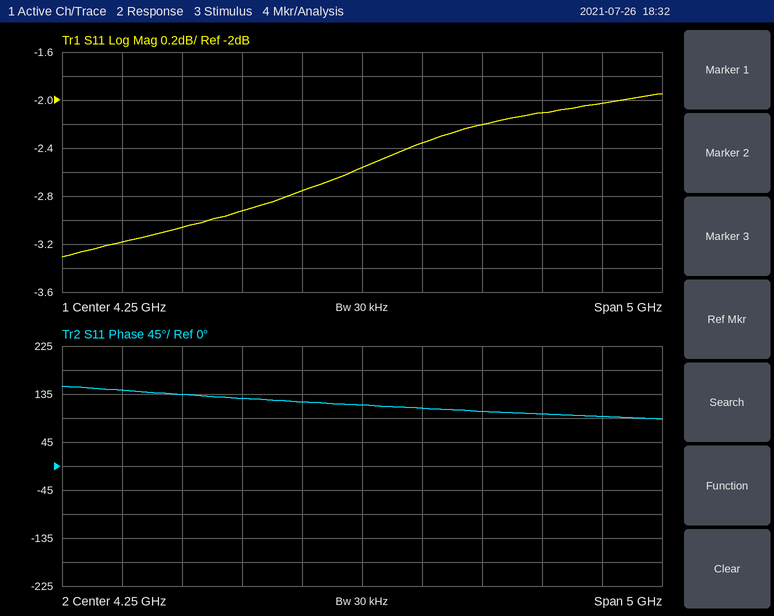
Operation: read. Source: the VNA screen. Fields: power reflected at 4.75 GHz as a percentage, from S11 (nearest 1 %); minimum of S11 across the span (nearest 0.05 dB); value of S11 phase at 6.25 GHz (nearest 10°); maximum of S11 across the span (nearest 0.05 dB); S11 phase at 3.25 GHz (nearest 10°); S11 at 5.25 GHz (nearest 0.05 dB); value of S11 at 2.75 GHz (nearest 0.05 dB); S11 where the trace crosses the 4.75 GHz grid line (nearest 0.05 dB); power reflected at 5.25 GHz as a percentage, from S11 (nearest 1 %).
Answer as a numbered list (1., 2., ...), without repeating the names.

1. 58 %
2. -3.30 dB
3. 90°
4. -1.95 dB
5. 130°
6. -2.20 dB
7. -3.05 dB
8. -2.35 dB
9. 60 %
